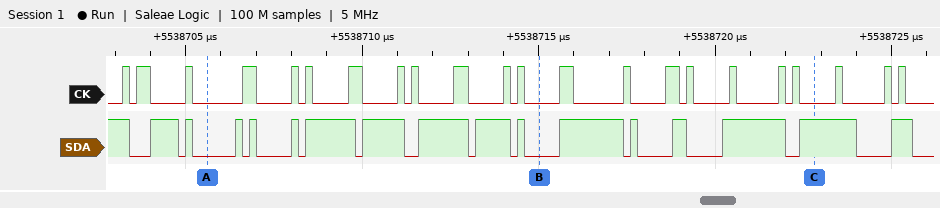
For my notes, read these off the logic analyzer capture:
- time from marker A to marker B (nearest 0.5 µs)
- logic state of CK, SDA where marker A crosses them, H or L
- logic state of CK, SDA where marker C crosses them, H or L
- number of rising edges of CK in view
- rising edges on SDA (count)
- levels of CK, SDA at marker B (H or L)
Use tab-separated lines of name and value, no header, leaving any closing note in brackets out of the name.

time from marker A to marker B	9.5 µs
logic state of CK, SDA where marker A crosses them, H or L	CK=L, SDA=L
logic state of CK, SDA where marker C crosses them, H or L	CK=L, SDA=H
number of rising edges of CK in view	22
rising edges on SDA	16
levels of CK, SDA at marker B	CK=L, SDA=L
